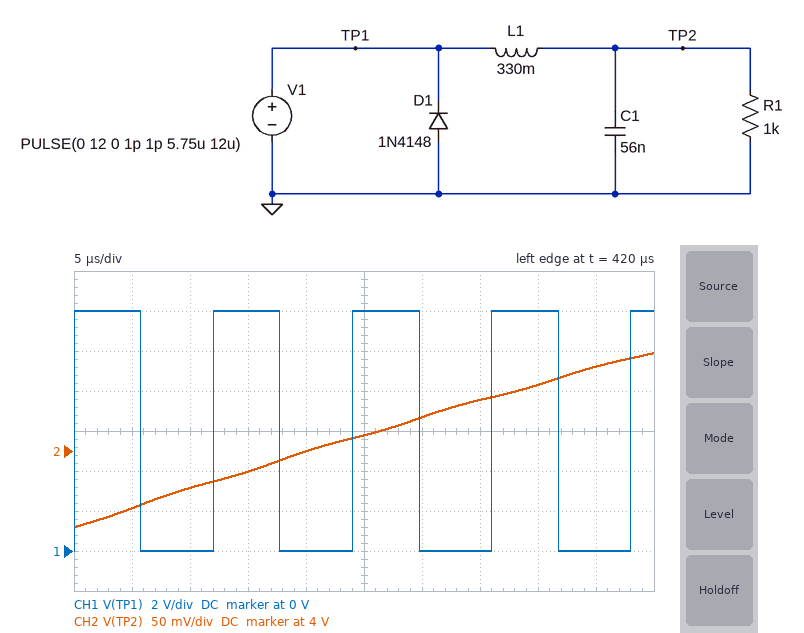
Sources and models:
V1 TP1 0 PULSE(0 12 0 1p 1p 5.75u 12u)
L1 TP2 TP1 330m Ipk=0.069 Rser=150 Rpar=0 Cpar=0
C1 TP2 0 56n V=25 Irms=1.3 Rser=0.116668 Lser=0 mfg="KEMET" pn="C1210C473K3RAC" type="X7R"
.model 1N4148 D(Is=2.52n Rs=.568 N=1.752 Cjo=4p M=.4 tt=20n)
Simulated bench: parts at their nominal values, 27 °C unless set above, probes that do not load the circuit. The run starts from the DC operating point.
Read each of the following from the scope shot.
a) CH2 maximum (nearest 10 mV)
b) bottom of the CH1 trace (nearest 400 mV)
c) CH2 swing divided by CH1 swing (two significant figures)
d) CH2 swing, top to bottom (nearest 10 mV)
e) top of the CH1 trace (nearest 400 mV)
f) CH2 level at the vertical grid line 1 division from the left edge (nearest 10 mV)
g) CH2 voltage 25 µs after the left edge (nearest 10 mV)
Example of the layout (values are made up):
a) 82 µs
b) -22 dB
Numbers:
a) 4.12 V
b) 0 V
c) 0.018
d) 220 mV
e) 12.0 V
f) 3.93 V
g) 4.02 V
